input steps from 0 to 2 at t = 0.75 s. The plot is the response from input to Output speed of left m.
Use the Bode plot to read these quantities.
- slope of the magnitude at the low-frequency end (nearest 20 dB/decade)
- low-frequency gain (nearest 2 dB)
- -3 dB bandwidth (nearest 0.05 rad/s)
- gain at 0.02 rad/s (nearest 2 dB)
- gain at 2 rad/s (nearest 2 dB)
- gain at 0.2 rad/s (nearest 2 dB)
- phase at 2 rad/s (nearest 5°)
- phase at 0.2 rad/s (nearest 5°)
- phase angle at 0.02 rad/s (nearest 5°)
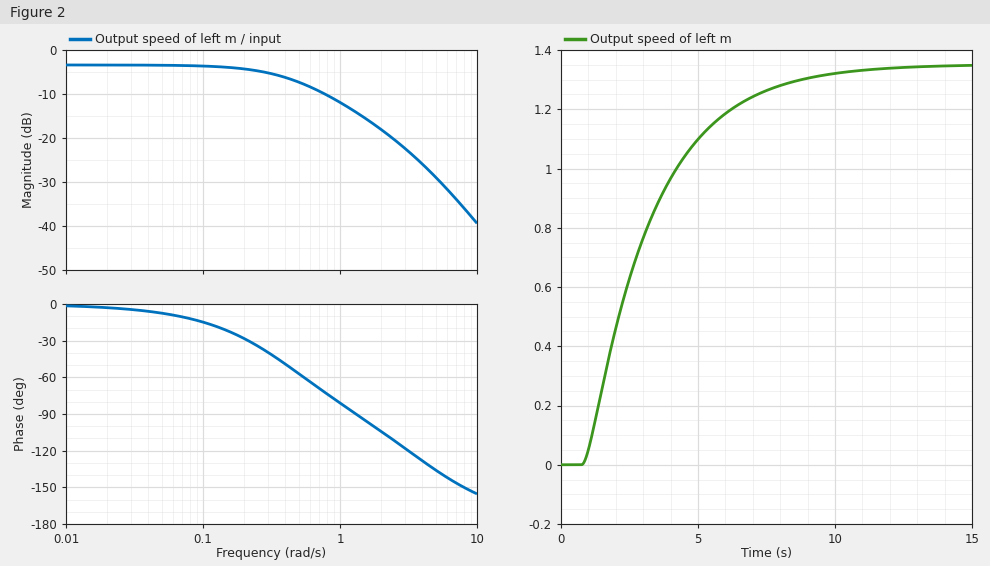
0 dB/decade
-4 dB
0.40 rad/s
-4 dB
-18 dB
-4 dB
-105°
-30°
-5°
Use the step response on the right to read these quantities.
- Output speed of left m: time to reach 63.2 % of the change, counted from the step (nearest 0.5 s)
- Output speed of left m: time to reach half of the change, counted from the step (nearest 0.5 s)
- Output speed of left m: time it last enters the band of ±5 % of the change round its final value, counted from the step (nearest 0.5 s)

2.5 s
2.0 s
7.5 s
